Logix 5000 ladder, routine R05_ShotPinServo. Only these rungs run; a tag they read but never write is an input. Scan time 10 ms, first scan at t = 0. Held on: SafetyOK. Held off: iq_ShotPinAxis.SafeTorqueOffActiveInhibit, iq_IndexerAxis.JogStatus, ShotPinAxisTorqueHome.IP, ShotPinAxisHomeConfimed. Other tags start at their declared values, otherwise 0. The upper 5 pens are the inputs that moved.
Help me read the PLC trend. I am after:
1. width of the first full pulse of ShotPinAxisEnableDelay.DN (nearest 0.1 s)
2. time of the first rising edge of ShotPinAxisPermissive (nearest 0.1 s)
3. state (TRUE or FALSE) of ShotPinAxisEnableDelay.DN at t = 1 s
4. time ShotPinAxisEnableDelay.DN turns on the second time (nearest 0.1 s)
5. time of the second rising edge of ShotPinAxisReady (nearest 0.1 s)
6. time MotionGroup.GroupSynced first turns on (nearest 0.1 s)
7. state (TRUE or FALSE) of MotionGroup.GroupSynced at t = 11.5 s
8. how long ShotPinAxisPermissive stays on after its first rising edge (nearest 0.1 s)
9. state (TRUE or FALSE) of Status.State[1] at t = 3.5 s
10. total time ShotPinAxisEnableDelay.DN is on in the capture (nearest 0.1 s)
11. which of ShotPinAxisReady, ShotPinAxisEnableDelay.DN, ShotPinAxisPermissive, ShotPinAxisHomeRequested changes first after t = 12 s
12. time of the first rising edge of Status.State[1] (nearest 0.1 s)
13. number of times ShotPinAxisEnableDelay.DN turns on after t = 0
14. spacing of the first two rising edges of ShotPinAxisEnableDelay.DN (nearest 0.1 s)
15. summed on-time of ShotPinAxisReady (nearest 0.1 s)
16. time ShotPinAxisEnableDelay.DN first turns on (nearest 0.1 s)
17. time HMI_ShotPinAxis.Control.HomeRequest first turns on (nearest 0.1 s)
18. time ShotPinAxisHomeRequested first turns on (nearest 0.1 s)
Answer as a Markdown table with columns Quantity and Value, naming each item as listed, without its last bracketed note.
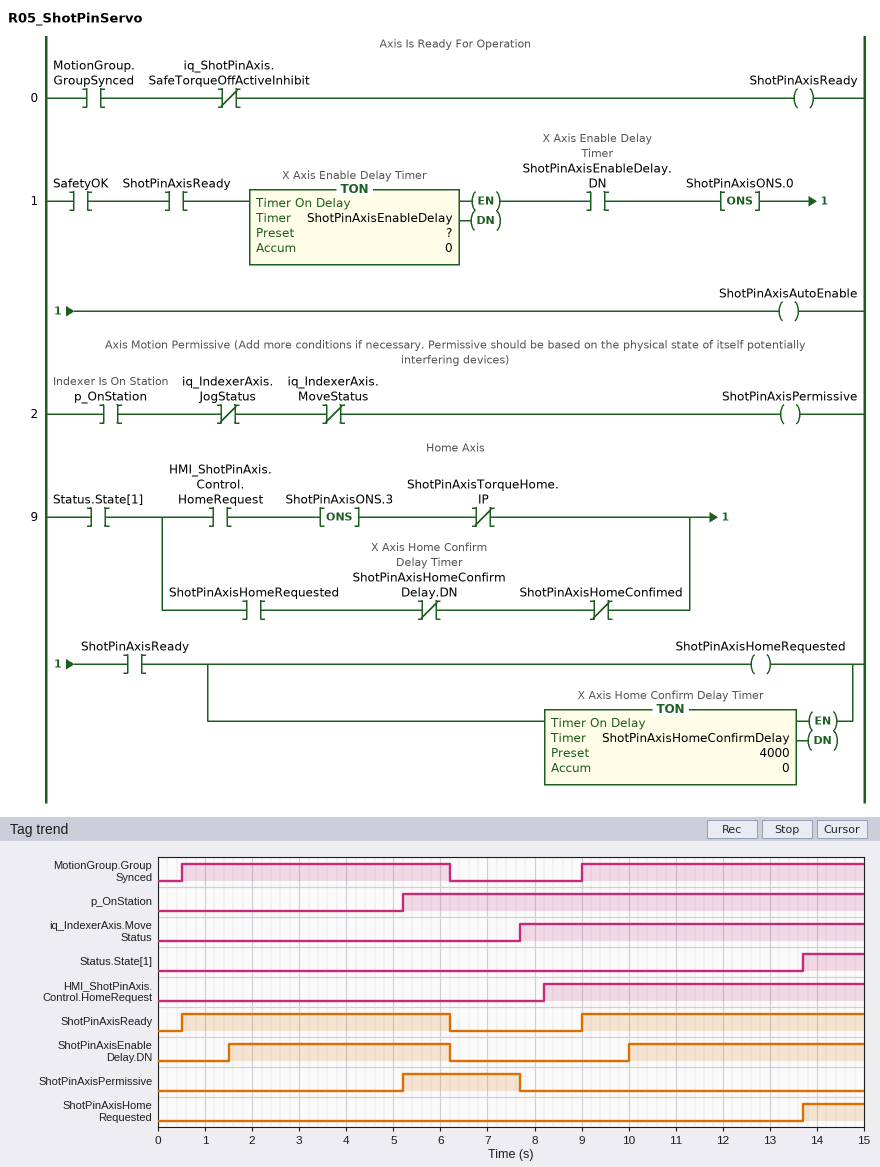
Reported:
| Quantity | Value |
|---|---|
| width of the first full pulse of ShotPinAxisEnableDelay.DN | 4.7 s |
| time of the first rising edge of ShotPinAxisPermissive | 5.2 s |
| state (TRUE or FALSE) of ShotPinAxisEnableDelay.DN at t = 1 s | FALSE |
| time ShotPinAxisEnableDelay.DN turns on the second time | 10.0 s |
| time of the second rising edge of ShotPinAxisReady | 9.0 s |
| time MotionGroup.GroupSynced first turns on | 0.5 s |
| state (TRUE or FALSE) of MotionGroup.GroupSynced at t = 11.5 s | TRUE |
| how long ShotPinAxisPermissive stays on after its first rising edge | 2.5 s |
| state (TRUE or FALSE) of Status.State[1] at t = 3.5 s | FALSE |
| total time ShotPinAxisEnableDelay.DN is on in the capture | 9.7 s |
| which of ShotPinAxisReady, ShotPinAxisEnableDelay.DN, ShotPinAxisPermissive, ShotPinAxisHomeRequested changes first after t = 12 s | ShotPinAxisHomeRequested |
| time of the first rising edge of Status.State[1] | 13.7 s |
| number of times ShotPinAxisEnableDelay.DN turns on after t = 0 | 2 |
| spacing of the first two rising edges of ShotPinAxisEnableDelay.DN | 8.5 s |
| summed on-time of ShotPinAxisReady | 11.7 s |
| time ShotPinAxisEnableDelay.DN first turns on | 1.5 s |
| time HMI_ShotPinAxis.Control.HomeRequest first turns on | 8.2 s |
| time ShotPinAxisHomeRequested first turns on | 13.7 s |
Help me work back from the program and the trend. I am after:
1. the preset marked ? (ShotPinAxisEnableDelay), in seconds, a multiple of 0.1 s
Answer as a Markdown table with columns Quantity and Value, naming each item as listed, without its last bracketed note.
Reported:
| Quantity | Value |
|---|---|
| the preset marked ? (ShotPinAxisEnableDelay), in seconds, a multiple of 0.1 s | 1.0 s |
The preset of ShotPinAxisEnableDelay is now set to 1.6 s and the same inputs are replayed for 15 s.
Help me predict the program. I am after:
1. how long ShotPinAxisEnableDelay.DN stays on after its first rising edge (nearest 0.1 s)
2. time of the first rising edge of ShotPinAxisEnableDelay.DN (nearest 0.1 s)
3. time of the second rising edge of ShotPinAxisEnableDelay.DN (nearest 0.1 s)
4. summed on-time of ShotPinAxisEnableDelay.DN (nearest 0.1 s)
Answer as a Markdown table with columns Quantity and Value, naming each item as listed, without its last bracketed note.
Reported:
| Quantity | Value |
|---|---|
| how long ShotPinAxisEnableDelay.DN stays on after its first rising edge | 4.1 s |
| time of the first rising edge of ShotPinAxisEnableDelay.DN | 2.1 s |
| time of the second rising edge of ShotPinAxisEnableDelay.DN | 10.6 s |
| summed on-time of ShotPinAxisEnableDelay.DN | 8.5 s |
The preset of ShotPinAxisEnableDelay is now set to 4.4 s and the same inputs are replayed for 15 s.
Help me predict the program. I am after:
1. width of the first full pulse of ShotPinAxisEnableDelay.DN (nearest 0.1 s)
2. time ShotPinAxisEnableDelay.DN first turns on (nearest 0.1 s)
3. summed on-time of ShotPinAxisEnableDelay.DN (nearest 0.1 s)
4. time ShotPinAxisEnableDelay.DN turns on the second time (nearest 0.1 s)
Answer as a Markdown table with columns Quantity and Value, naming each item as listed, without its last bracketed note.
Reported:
| Quantity | Value |
|---|---|
| width of the first full pulse of ShotPinAxisEnableDelay.DN | 1.3 s |
| time ShotPinAxisEnableDelay.DN first turns on | 4.9 s |
| summed on-time of ShotPinAxisEnableDelay.DN | 2.9 s |
| time ShotPinAxisEnableDelay.DN turns on the second time | 13.4 s |
